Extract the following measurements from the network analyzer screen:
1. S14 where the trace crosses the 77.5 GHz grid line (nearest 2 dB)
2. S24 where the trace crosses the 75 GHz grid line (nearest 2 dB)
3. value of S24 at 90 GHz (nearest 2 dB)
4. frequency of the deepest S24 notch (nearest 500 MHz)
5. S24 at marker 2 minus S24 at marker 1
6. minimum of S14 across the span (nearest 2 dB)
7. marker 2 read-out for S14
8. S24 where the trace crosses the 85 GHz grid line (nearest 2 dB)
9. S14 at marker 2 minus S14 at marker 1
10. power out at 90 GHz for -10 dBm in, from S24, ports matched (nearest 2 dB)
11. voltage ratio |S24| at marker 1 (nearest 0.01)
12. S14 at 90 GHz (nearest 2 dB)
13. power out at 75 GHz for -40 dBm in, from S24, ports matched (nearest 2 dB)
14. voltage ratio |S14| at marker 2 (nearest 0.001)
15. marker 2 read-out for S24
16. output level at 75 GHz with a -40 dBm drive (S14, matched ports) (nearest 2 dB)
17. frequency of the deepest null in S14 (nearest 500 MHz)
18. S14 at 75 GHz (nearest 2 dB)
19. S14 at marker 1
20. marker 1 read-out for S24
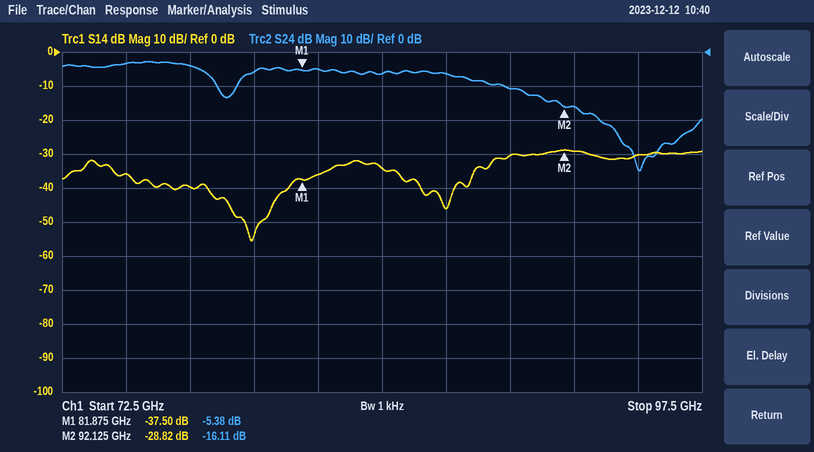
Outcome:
-40 dB
-4 dB
-10 dB
95.0 GHz
-10.73 dB
-56 dB
-28.82 dB
-6 dB
8.68 dB
-20 dBm
0.54
-30 dB
-44 dBm
0.036
-16.11 dB
-76 dBm
80.0 GHz
-36 dB
-37.50 dB
-5.38 dB
